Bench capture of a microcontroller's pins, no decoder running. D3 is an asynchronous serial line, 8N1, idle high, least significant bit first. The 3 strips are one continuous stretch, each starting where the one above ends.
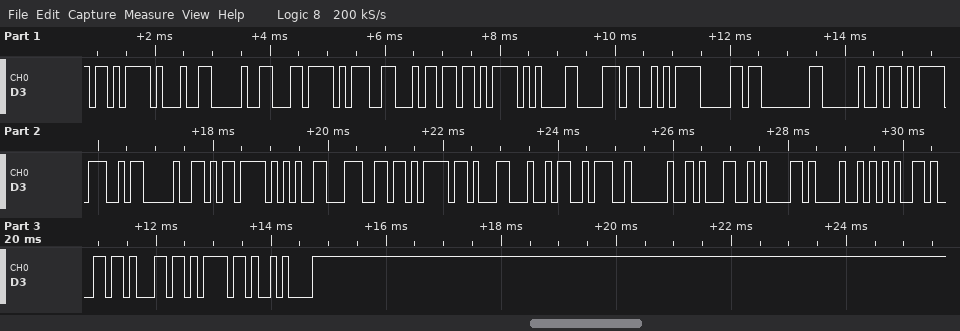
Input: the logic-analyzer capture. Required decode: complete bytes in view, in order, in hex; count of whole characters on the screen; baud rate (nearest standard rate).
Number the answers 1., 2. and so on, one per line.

1. EB 91 90 EC 9D B4 EB 85 B8 EA B0 80 20 EB A7 90 ED 95 9C EB 8B A4 3A 20 31 61 48 65 6C 6C 6F 0A
2. 32
3. 9600 baud
